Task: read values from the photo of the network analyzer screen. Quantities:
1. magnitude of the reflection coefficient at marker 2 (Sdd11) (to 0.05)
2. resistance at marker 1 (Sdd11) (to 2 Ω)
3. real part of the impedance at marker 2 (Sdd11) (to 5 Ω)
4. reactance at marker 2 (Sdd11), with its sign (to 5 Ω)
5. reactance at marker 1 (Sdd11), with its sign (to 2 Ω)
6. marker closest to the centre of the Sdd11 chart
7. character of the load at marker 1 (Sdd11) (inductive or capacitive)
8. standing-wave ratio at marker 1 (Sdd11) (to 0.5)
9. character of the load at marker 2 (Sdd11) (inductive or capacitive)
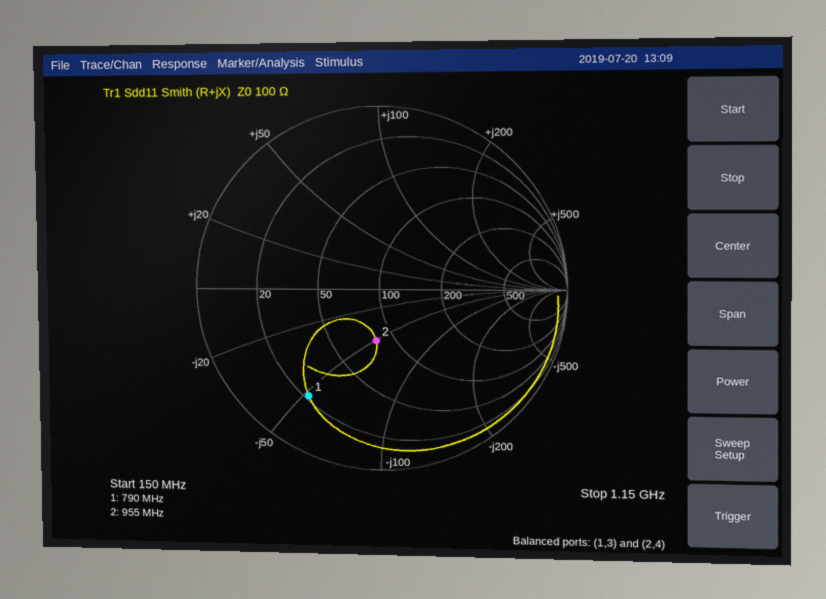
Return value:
0.30
22 Ω
80 Ω
-50 Ω
-52 Ω
marker 2
capacitive
6.0
capacitive
